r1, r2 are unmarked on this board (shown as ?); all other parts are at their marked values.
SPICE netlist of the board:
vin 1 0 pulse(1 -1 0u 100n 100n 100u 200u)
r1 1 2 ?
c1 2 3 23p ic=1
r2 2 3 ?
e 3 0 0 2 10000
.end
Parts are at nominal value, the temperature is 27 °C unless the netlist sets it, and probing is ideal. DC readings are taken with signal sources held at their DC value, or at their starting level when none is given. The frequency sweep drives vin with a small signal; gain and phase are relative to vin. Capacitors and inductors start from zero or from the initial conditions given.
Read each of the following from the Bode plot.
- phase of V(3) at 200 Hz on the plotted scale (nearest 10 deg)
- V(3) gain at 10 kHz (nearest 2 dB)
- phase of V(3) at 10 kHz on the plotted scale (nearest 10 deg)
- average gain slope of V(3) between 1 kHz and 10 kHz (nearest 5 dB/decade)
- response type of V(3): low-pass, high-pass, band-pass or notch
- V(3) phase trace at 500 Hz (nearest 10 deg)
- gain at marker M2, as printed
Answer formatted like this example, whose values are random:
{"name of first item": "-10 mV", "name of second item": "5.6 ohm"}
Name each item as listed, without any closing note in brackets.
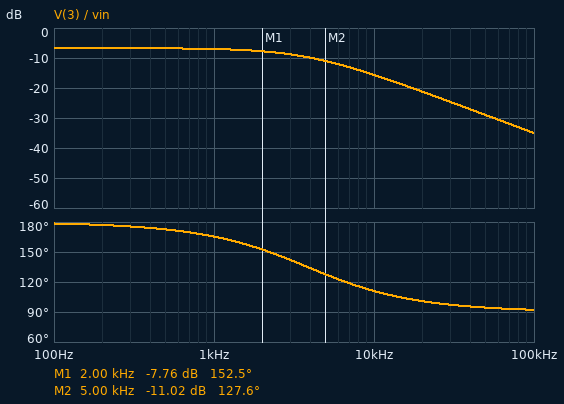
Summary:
{"phase of V(3) at 200 Hz on the plotted scale": "180 deg", "V(3) gain at 10 kHz": "-16 dB", "phase of V(3) at 10 kHz on the plotted scale": "110 deg", "average gain slope of V(3) between 1 kHz and 10 kHz": "-10 dB/decade", "response type of V(3): low-pass, high-pass, band-pass or notch": "low-pass", "V(3) phase trace at 500 Hz": "170 deg", "gain at marker M2, as printed": "-11.02 dB"}
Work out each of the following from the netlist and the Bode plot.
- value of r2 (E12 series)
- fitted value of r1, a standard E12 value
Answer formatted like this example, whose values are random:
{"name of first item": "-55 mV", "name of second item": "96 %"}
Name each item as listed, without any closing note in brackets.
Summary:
{"value of r2": "1.8 MΩ", "fitted value of r1, a standard E12 value": "3.9 MΩ"}
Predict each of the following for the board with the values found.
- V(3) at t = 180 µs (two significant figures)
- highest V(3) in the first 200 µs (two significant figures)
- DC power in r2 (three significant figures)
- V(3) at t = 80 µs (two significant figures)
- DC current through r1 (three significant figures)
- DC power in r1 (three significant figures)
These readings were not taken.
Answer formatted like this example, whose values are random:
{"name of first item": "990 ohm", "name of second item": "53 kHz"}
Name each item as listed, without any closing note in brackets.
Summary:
{"V(3) at t = 180 µs": "-350 mV", "highest V(3) in the first 200 µs": "330 mV", "DC power in r2": "118 nW", "V(3) at t = 80 µs": "250 mV", "DC current through r1": "256 nA", "DC power in r1": "256 nW"}
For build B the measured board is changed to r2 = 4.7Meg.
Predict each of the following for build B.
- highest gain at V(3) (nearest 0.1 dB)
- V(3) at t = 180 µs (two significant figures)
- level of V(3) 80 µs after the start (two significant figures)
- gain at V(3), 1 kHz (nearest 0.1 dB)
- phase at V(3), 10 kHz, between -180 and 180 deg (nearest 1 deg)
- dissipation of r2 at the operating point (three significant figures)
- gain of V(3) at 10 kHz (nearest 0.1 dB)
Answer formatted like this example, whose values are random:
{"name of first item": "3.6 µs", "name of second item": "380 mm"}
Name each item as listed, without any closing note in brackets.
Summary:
{"highest gain at V(3)": "1.6 dB", "V(3) at t = 180 µs": "-470 mV", "level of V(3) 80 µs after the start": "150 mV", "gain at V(3), 1 kHz": "0 dB", "phase at V(3), 10 kHz, between -180 and 180 deg": "98 deg", "dissipation of r2 at the operating point": "309 nW", "gain of V(3) at 10 kHz": "-15.1 dB"}
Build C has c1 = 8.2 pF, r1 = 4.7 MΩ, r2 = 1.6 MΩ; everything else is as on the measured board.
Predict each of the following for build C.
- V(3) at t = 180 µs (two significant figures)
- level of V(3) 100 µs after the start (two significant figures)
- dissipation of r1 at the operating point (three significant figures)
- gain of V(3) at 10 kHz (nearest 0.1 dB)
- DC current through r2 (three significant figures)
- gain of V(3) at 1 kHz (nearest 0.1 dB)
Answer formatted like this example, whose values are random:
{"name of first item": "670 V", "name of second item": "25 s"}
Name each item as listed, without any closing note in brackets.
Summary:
{"V(3) at t = 180 µs": "-340 mV", "level of V(3) 100 µs after the start": "340 mV", "dissipation of r1 at the operating point": "213 nW", "gain of V(3) at 10 kHz": "-11.6 dB", "DC current through r2": "213 nA", "gain of V(3) at 1 kHz": "-9.4 dB"}
